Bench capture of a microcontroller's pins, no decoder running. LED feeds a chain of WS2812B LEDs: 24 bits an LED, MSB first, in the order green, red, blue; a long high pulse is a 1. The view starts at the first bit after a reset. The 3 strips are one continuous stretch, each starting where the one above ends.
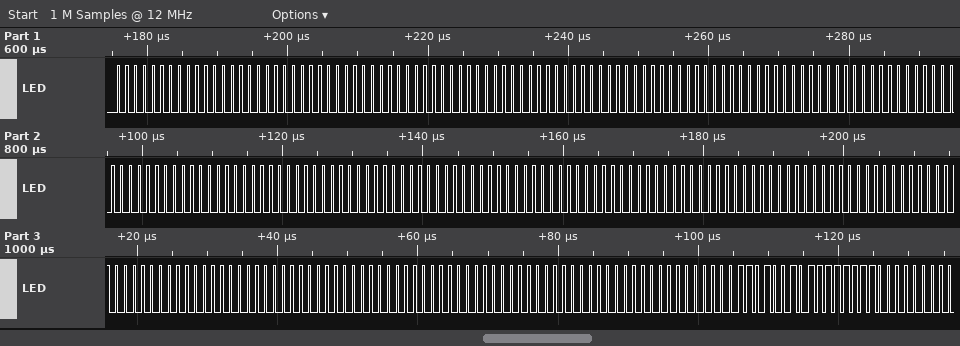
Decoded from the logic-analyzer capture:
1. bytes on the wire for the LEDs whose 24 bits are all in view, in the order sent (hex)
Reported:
00 00 00 00 00 00 00 00 00 00 00 00 00 00 00 00 00 00 00 00 00 00 00 00 00 00 00 00 00 00 00 00 00 D2 FF 00
